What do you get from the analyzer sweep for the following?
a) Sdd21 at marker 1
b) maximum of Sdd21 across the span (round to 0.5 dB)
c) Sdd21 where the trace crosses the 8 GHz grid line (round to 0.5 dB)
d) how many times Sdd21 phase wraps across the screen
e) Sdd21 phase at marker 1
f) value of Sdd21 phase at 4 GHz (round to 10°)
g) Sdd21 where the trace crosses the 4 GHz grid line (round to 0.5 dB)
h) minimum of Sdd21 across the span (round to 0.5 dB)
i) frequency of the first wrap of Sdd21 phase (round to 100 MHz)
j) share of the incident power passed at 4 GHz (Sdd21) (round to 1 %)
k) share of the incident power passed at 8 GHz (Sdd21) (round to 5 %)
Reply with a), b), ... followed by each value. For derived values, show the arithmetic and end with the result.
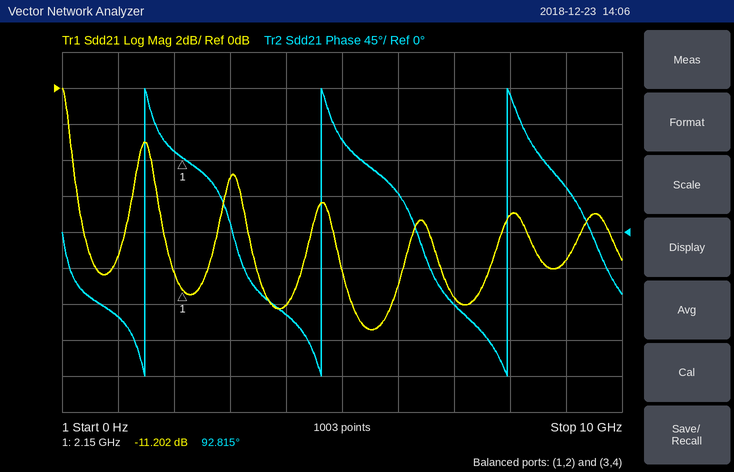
a) -11.202 dB
b) 0.0 dB
c) -7.0 dB
d) 3
e) 92.815°
f) -100°
g) -12.0 dB
h) -13.5 dB
i) 1.5 GHz
j) 10^(-12/10) ≈ 6 %
k) 10^(-7/10) ≈ 20 %
